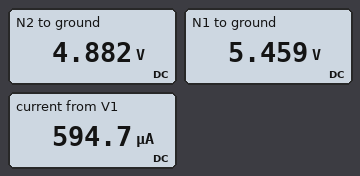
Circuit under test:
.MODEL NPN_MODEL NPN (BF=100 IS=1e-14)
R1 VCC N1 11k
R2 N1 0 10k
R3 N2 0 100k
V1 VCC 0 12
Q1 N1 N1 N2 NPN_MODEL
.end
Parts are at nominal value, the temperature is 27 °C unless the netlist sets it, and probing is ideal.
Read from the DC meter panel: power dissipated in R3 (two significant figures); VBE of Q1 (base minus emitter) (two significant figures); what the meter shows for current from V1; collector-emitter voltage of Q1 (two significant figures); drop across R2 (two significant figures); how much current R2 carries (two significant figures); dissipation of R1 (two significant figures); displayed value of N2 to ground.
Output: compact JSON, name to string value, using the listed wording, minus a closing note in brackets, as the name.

{"power dissipated in R3": "240 µW", "VBE of Q1 (base minus emitter)": "580 mV", "what the meter shows for current from V1": "594.7 µA", "collector-emitter voltage of Q1": "580 mV", "drop across R2": "5.5 V", "how much current R2 carries": "550 µA", "dissipation of R1": "3.9 mW", "displayed value of N2 to ground": "4.882 V"}
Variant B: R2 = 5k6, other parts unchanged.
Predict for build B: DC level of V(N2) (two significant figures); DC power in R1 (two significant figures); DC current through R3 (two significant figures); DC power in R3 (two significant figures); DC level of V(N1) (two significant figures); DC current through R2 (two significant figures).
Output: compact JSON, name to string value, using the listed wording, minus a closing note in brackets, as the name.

{"DC level of V(N2)": "3.4 V", "DC power in R1": "5.9 mW", "DC current through R3": "34 µA", "DC power in R3": "110 µW", "DC level of V(N1)": "3.9 V", "DC current through R2": "700 µA"}
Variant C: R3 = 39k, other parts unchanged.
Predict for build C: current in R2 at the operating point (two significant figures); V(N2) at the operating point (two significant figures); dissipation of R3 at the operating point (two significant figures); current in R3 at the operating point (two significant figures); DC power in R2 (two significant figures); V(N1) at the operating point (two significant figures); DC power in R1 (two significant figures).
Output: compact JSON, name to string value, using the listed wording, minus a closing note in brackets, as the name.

{"current in R2 at the operating point": "510 µA", "V(N2) at the operating point": "4.5 V", "dissipation of R3 at the operating point": "520 µW", "current in R3 at the operating point": "120 µA", "DC power in R2": "2.6 mW", "V(N1) at the operating point": "5.1 V", "DC power in R1": "4.3 mW"}
